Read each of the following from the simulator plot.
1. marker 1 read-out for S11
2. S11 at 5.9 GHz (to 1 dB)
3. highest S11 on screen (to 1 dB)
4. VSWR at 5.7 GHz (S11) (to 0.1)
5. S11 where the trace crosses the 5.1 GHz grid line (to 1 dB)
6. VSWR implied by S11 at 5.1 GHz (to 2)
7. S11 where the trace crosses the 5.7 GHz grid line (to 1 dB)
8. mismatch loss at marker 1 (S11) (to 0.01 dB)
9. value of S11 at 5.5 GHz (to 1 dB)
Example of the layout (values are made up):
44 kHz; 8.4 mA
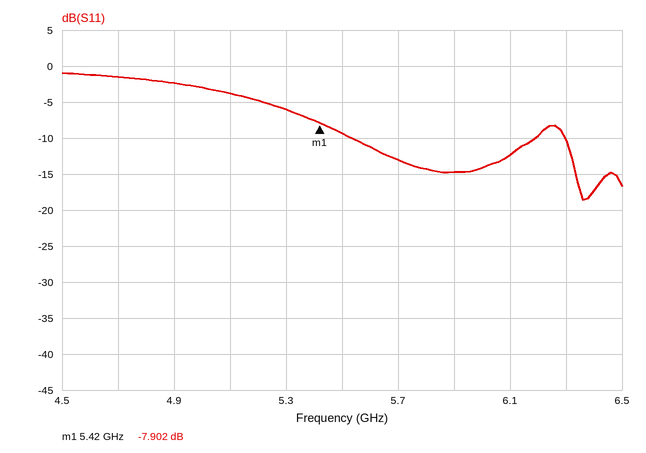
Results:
-7.902 dB; -15 dB; -1 dB; 1.6; -4 dB; 4; -13 dB; 0.77 dB; -9 dB
